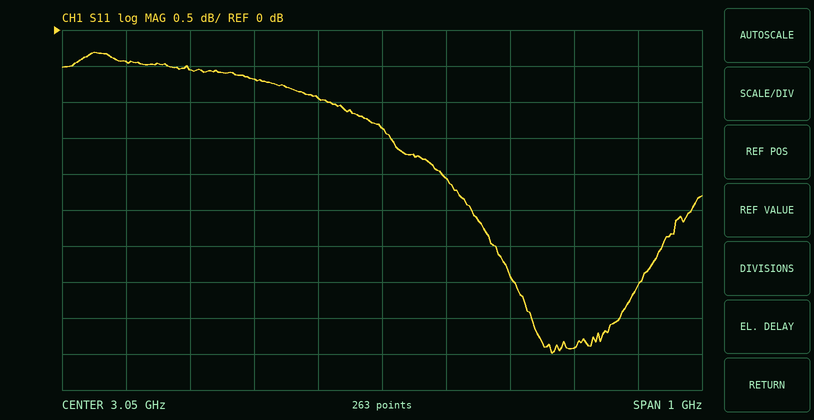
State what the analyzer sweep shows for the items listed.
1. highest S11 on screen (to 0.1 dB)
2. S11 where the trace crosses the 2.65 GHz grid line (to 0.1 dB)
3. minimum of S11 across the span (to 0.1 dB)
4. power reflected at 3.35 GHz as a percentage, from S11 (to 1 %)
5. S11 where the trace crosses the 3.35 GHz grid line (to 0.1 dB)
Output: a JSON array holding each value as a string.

["-0.3 dB", "-0.4 dB", "-4.5 dB", "36 %", "-4.4 dB"]
